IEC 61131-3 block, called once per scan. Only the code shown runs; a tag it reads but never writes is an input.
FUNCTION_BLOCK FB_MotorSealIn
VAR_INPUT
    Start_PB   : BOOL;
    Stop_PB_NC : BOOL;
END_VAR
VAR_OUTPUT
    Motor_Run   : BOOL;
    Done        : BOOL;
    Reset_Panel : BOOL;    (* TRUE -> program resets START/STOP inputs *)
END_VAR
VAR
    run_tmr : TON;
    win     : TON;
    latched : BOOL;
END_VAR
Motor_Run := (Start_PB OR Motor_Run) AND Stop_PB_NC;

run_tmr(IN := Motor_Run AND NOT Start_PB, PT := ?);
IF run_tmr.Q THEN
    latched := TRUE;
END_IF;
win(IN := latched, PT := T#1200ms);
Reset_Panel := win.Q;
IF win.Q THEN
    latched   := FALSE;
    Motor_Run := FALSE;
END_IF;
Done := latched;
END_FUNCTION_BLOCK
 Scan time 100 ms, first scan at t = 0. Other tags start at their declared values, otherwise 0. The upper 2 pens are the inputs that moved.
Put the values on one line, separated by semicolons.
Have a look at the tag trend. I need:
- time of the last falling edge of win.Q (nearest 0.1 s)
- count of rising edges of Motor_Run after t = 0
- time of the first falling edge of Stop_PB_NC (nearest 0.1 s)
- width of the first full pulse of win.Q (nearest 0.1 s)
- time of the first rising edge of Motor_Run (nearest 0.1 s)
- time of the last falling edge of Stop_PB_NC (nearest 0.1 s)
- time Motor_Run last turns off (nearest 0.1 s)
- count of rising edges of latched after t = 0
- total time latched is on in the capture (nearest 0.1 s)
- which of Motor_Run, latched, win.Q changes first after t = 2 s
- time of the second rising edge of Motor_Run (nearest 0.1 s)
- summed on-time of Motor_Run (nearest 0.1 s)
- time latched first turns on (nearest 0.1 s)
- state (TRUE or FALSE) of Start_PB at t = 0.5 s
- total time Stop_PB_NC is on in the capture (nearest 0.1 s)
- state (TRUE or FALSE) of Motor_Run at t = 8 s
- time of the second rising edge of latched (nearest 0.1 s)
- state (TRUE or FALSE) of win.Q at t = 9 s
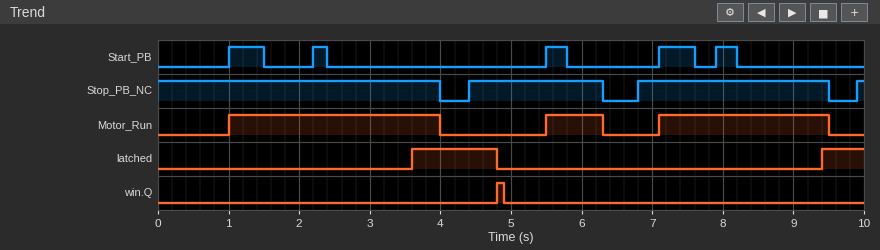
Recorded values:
4.9 s; 3; 4.0 s; 0.1 s; 1.0 s; 9.5 s; 9.5 s; 2; 1.8 s; latched; 5.5 s; 6.2 s; 3.6 s; FALSE; 8.7 s; TRUE; 9.4 s; FALSE
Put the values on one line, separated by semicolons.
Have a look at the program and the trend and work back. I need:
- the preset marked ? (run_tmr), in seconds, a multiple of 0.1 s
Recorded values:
1.2 s
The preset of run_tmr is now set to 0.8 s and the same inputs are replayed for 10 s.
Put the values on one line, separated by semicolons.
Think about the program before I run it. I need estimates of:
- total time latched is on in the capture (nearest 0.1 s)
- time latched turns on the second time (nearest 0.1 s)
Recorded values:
2.2 s; 9.0 s
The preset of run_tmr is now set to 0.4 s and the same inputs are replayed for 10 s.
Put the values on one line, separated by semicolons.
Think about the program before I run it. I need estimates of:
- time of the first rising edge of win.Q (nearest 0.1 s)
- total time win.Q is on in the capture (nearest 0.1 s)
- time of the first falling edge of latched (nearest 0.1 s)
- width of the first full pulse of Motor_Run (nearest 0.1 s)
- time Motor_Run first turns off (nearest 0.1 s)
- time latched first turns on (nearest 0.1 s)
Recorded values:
3.1 s; 0.3 s; 3.1 s; 2.1 s; 3.1 s; 1.9 s
